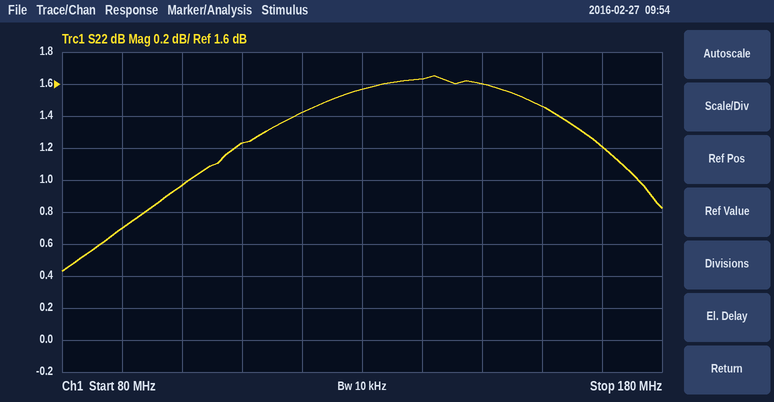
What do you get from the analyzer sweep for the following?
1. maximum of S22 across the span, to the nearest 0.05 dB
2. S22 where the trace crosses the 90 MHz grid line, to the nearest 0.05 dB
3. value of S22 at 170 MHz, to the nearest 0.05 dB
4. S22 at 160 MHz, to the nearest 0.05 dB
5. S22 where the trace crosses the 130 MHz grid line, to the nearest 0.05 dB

1.65 dB
0.70 dB
1.20 dB
1.45 dB
1.55 dB
